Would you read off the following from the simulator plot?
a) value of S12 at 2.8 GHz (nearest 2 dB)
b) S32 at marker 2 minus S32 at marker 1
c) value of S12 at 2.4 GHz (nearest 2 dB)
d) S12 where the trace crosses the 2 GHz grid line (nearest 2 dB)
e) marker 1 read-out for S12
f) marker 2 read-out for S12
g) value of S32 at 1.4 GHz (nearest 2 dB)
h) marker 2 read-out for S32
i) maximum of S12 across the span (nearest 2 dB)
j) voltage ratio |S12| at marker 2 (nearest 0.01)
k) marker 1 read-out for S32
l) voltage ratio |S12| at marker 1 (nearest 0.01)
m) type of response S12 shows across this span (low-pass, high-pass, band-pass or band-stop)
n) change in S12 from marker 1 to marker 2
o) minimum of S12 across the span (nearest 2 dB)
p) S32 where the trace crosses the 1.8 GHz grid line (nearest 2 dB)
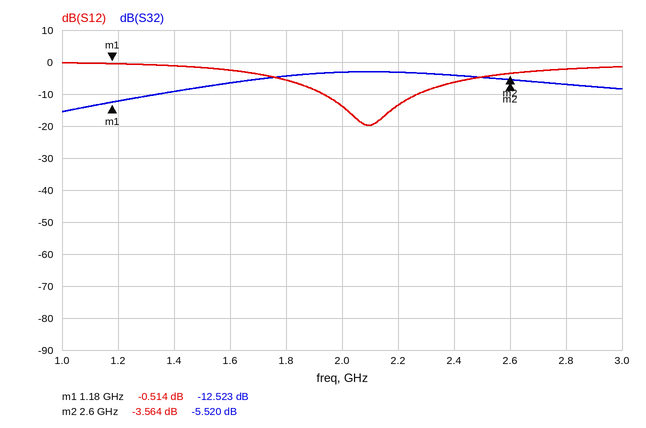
-2 dB
7.003 dB
-6 dB
-14 dB
-0.514 dB
-3.564 dB
-10 dB
-5.520 dB
0 dB
0.66
-12.523 dB
0.94
band-stop
-3.050 dB
-20 dB
-4 dB
